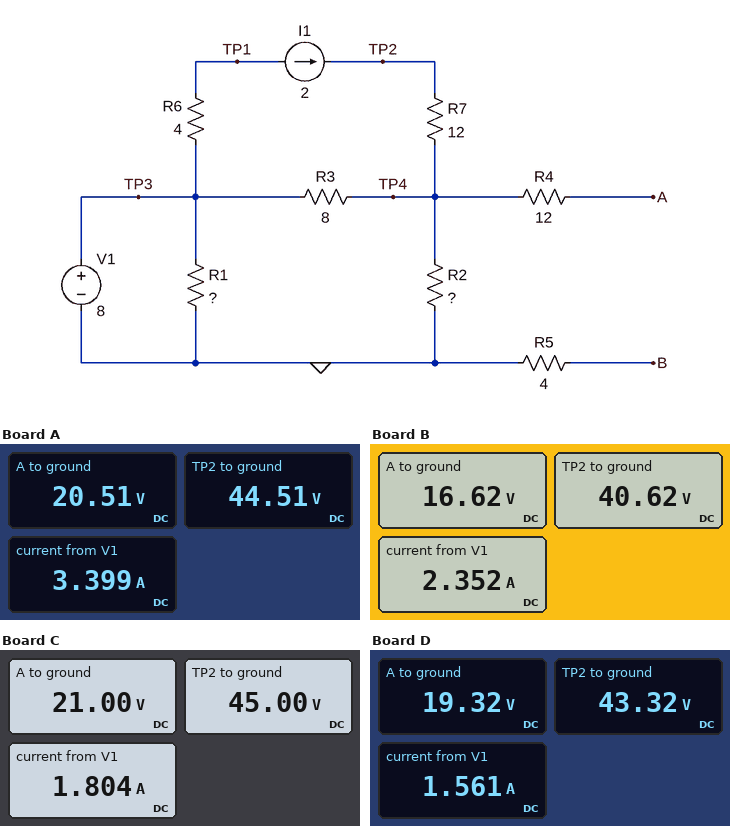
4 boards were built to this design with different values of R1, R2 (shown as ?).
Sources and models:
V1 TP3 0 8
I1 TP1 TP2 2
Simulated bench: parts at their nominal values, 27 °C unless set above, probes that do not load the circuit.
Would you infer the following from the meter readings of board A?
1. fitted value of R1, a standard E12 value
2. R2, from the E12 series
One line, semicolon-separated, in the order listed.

2.7 Ω; 47 Ω
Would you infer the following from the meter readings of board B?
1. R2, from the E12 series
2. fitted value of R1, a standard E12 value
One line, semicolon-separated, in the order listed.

18 Ω; 5.6 Ω
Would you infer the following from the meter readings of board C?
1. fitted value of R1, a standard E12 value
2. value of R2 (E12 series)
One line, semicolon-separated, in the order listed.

5.6 Ω; 56 Ω
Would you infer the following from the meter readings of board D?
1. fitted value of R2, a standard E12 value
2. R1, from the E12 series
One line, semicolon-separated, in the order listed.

33 Ω; 8.2 Ω
